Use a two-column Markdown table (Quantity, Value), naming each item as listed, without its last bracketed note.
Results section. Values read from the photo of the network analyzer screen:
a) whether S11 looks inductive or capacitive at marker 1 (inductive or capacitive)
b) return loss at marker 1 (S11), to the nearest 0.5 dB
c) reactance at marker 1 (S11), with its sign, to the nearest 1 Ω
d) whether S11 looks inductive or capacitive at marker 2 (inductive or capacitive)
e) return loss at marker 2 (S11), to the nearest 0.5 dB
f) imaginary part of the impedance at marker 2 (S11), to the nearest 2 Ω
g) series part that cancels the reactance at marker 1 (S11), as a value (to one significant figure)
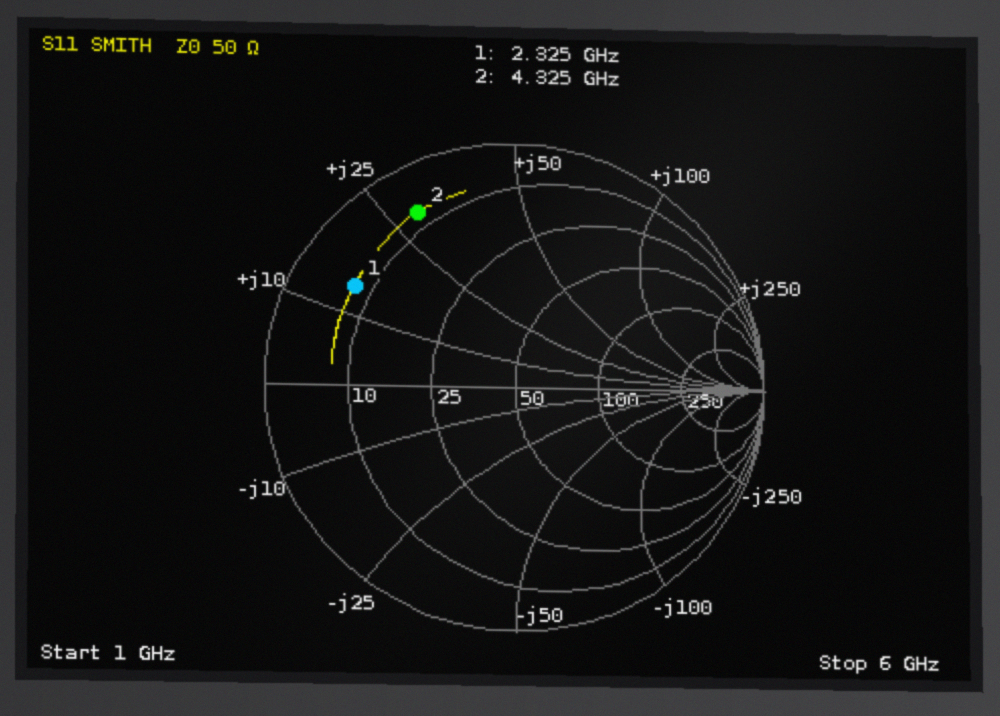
| Quantity | Value |
|---|---|
| whether S11 looks inductive or capacitive at marker 1 | inductive |
| return loss at marker 1 (S11), to the nearest 0.5 dB | 2.5 dB |
| reactance at marker 1 (S11), with its sign, to the nearest 1 Ω | +14 Ω |
| whether S11 looks inductive or capacitive at marker 2 | inductive |
| return loss at marker 2 (S11), to the nearest 0.5 dB | 2.0 dB |
| imaginary part of the impedance at marker 2 (S11), to the nearest 2 Ω | +30 Ω |
| series part that cancels the reactance at marker 1 (S11), as a value | 5 pF |
